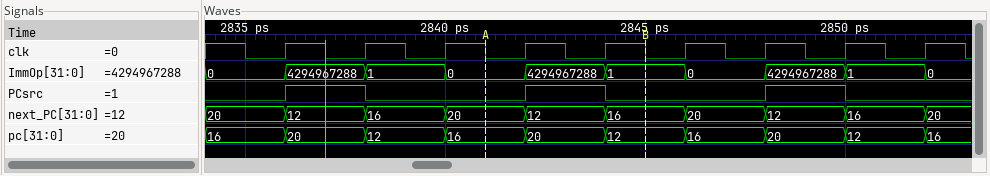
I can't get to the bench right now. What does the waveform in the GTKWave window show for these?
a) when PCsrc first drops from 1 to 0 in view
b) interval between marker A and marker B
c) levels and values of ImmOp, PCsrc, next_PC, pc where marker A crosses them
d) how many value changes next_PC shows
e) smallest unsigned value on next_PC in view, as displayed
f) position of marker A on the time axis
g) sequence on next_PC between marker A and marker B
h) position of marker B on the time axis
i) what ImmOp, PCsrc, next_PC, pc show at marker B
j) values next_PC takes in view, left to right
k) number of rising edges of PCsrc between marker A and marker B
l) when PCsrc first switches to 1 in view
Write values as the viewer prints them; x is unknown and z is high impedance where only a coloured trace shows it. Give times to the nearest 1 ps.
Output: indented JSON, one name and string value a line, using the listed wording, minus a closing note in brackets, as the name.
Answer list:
{
  "when PCsrc first drops from 1 to 0 in view": "2838 ps",
  "interval between marker A and marker B": "4 ps",
  "levels and values of ImmOp, PCsrc, next_PC, pc where marker A crosses them": "ImmOp=0, PCsrc=0, next_PC=20, pc=16",
  "how many value changes next_PC shows": "9",
  "smallest unsigned value on next_PC in view, as displayed": "12",
  "position of marker A on the time axis": "2841 ps",
  "sequence on next_PC between marker A and marker B": "20, 12, 16",
  "position of marker B on the time axis": "2845 ps",
  "what ImmOp, PCsrc, next_PC, pc show at marker B": "ImmOp=1, PCsrc=0, next_PC=16, pc=12",
  "values next_PC takes in view, left to right": "20, 12, 16, 20, 12, 16, 20, 12, 16, 20",
  "number of rising edges of PCsrc between marker A and marker B": "1",
  "when PCsrc first switches to 1 in view": "2836 ps"
}
